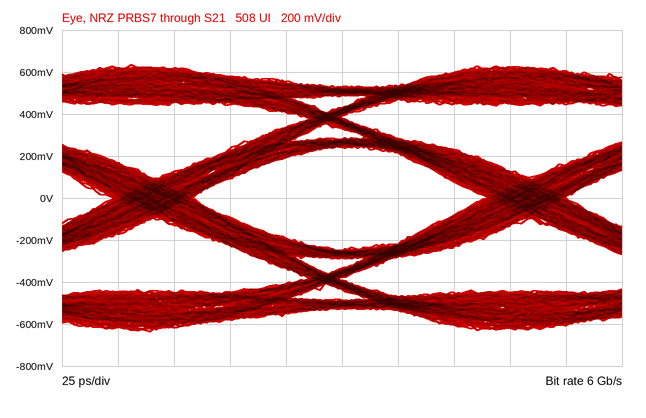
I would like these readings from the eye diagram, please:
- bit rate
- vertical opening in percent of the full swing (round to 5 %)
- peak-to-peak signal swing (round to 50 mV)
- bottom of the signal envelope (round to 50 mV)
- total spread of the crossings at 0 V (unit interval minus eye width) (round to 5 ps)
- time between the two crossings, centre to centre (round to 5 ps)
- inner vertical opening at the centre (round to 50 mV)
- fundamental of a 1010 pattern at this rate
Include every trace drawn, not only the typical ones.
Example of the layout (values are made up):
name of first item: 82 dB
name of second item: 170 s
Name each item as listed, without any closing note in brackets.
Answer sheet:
bit rate: 6 Gb/s
vertical opening in percent of the full swing: 40 %
peak-to-peak signal swing: 1.25 V
bottom of the signal envelope: -650 mV
total spread of the crossings at 0 V (unit interval minus eye width): 35 ps
time between the two crossings, centre to centre: 165 ps
inner vertical opening at the centre: 500 mV
fundamental of a 1010 pattern at this rate: 3 GHz
